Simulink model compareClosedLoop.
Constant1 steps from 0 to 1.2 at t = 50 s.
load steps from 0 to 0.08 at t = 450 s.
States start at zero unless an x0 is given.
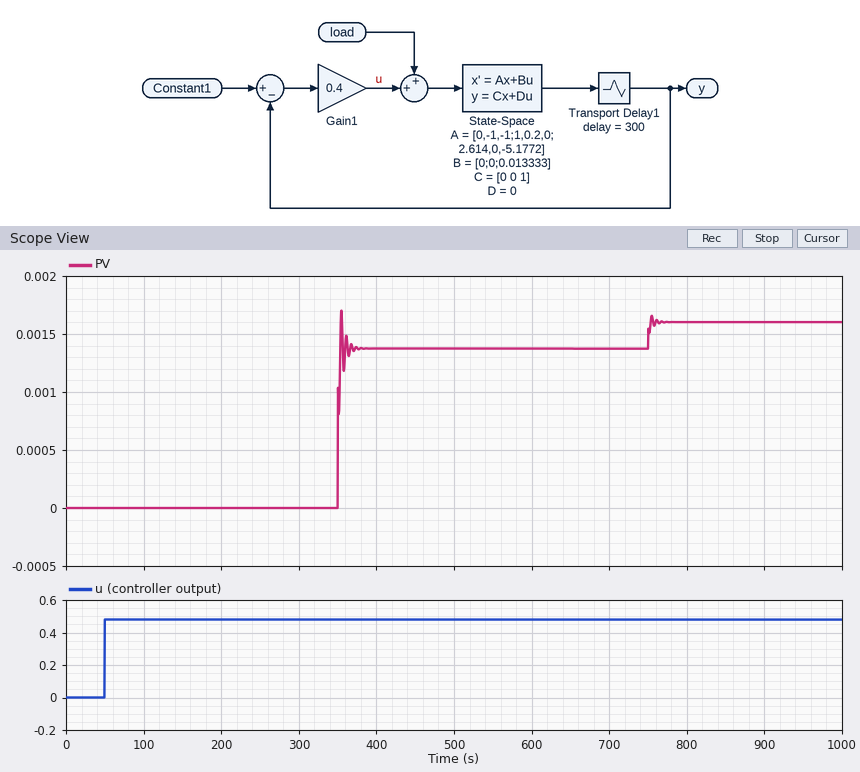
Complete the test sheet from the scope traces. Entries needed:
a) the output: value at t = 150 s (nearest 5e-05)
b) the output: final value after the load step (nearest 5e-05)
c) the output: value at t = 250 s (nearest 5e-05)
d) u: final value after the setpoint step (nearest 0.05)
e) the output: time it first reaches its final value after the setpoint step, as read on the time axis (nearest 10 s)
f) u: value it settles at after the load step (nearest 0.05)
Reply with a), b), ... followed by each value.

a) 0.00000
b) 0.00160
c) 0.00000
d) 0.50
e) 350 s
f) 0.50
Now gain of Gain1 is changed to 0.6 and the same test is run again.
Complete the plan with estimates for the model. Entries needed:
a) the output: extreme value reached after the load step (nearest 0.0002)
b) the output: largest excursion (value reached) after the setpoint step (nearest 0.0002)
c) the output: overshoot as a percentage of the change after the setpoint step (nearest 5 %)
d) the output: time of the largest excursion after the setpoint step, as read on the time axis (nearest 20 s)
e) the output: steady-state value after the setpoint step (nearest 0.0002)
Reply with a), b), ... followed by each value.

a) 0.0024
b) 0.0026
c) 25 %
d) 360 s
e) 0.0020
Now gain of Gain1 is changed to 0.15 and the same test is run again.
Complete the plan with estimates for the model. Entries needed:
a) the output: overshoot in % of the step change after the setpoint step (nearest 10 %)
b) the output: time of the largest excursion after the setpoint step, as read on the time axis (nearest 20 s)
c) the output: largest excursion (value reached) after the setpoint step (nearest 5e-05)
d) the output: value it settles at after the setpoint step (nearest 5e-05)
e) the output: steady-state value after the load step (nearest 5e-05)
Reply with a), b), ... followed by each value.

a) 20 %
b) 360 s
c) 0.00065
d) 0.00050
e) 0.00075
